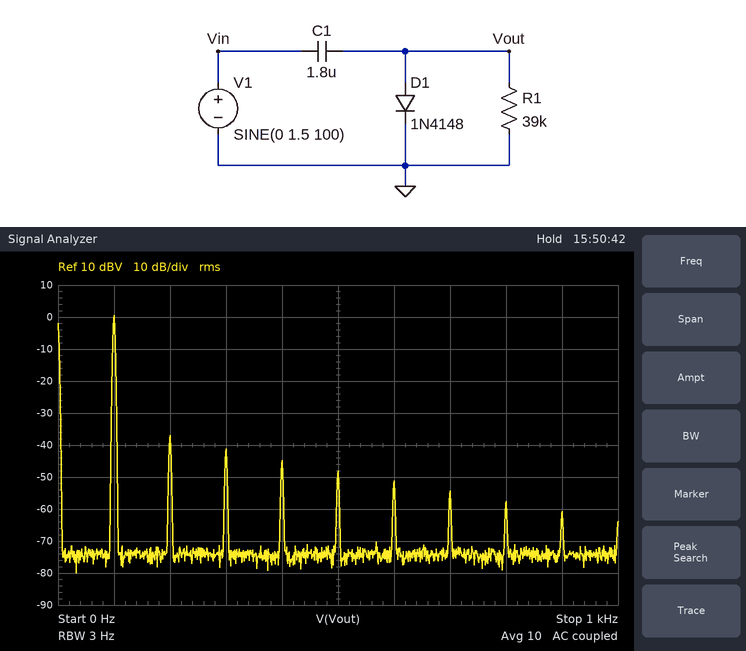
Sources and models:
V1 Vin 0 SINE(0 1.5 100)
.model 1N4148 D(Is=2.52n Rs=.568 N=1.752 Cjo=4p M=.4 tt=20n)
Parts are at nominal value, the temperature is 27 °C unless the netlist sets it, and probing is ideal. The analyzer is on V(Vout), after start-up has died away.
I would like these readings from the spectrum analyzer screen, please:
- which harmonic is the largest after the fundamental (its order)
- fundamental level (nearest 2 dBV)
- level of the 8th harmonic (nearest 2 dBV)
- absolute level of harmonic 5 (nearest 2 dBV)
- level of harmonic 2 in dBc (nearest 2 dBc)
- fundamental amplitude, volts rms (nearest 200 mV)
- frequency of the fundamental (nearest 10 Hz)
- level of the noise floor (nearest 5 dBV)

2
0 dBV
-58 dBV
-48 dBV
-38 dBc
1.0 V
100 Hz
-75 dBV
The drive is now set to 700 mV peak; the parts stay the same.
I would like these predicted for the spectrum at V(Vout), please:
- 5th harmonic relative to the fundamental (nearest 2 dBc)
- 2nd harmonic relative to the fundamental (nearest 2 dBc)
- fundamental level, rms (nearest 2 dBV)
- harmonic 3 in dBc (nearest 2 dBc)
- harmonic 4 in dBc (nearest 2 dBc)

-58 dBc
-44 dBc
-6 dBV
-48 dBc
-52 dBc
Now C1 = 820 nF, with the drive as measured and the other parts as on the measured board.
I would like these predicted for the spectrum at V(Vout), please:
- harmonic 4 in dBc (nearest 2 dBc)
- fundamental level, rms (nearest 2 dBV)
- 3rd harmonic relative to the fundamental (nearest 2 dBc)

-40 dBc
0 dBV
-36 dBc
